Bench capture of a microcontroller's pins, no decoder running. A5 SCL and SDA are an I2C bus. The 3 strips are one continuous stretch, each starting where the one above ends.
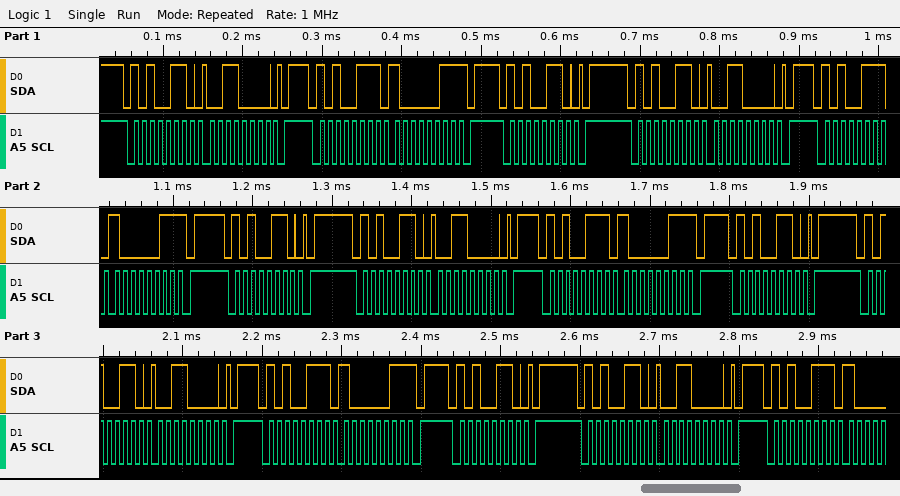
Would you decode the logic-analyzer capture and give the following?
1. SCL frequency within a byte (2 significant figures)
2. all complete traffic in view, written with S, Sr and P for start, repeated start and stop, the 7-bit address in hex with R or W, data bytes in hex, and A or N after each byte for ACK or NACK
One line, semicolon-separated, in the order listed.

100 kHz; S 53W A 30 A P S 53R A 83 N P S 53W A P S 53W A 30 A P S 53R A 83 N P S 53W A P S 53W A 30 A P S 53R A 83 N P S 53W A P S 53W A 30 A P S 53R A 83 N P S 53W A P S 53W A 30 A P S 53R A
